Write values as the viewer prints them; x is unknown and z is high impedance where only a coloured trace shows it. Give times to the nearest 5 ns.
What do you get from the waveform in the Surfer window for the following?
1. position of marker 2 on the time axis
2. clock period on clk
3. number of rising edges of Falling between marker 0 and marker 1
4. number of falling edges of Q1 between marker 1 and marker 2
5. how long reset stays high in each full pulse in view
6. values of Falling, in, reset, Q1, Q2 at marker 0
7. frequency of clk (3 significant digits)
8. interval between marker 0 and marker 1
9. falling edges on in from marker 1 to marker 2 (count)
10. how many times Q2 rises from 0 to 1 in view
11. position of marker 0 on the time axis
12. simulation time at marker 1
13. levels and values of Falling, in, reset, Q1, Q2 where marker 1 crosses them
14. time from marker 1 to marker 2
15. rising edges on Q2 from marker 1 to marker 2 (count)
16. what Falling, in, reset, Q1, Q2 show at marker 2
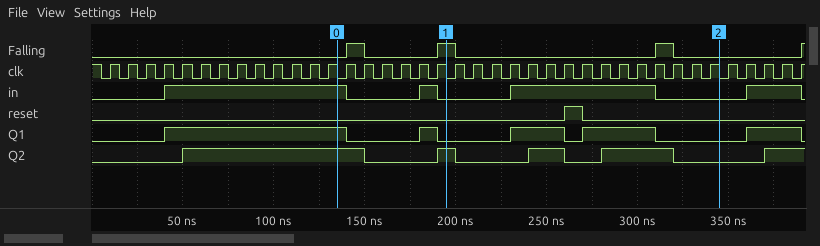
345 ns
10 ns
2
2
10 ns
Falling=0, in=1, reset=0, Q1=1, Q2=1
100 MHz
60 ns
1
5
135 ns
195 ns
Falling=1, in=0, reset=0, Q1=0, Q2=1
150 ns
2
Falling=0, in=0, reset=0, Q1=0, Q2=0
